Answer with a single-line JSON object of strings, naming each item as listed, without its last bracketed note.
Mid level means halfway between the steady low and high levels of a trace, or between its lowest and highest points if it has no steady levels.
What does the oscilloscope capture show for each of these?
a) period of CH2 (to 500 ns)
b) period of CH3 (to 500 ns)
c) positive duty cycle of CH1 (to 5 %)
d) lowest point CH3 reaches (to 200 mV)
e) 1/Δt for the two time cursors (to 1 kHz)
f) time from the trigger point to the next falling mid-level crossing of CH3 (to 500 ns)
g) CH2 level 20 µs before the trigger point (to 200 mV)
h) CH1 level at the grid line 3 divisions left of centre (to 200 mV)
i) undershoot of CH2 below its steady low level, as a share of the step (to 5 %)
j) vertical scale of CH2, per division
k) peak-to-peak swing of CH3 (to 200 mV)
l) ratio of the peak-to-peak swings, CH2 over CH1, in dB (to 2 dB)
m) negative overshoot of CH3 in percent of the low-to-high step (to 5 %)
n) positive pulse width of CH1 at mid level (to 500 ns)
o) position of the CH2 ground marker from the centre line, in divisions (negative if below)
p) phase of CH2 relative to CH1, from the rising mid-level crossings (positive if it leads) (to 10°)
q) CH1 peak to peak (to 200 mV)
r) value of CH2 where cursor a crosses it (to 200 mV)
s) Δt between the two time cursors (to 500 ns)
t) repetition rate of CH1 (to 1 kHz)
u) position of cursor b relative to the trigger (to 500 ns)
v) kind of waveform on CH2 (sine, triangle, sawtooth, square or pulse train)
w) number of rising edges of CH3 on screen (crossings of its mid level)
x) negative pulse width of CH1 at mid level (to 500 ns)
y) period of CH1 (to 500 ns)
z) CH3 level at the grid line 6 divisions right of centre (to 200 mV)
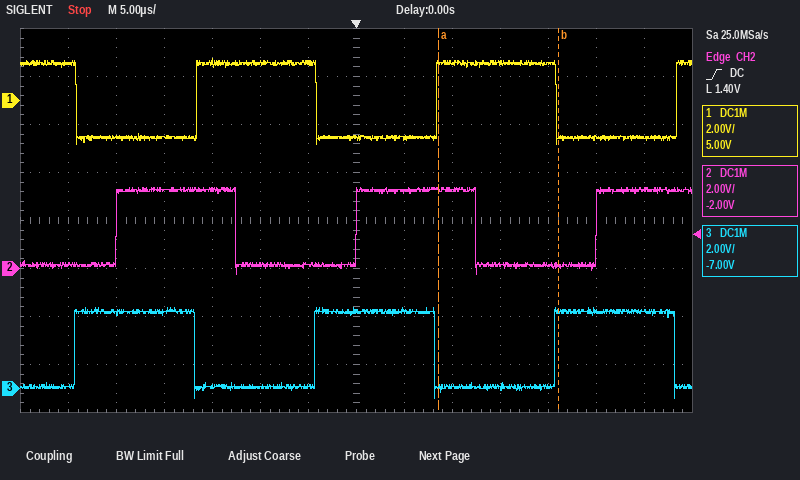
{"period of CH2": "25.0 µs", "period of CH3": "25.0 µs", "positive duty cycle of CH1": "50 %", "lowest point CH3 reaches": "-400 mV", "1/Δt for the two time cursors": "80 kHz", "time from the trigger point to the next falling mid-level crossing of CH3": "8.0 µs", "CH2 level 20 µs before the trigger point": "3.2 V", "CH1 level at the grid line 3 divisions left of centre": "1.6 V", "undershoot of CH2 below its steady low level, as a share of the step": "10 %", "vertical scale of CH2, per division": "2 V", "peak-to-peak swing of CH3": "3.8 V", "ratio of the peak-to-peak swings, CH2 over CH1, in dB": "0 dB", "negative overshoot of CH3 in percent of the low-to-high step": "15 %", "positive pulse width of CH1 at mid level": "12.5 µs", "position of the CH2 ground marker from the centre line, in divisions": "-1.0 div", "phase of CH2 relative to CH1, from the rising mid-level crossings (positive if it leads)": "+120°", "CH1 peak to peak": "3.6 V", "value of CH2 where cursor a crosses it": "3.2 V", "Δt between the two time cursors": "12.5 µs", "repetition rate of CH1": "40 kHz", "position of cursor b relative to the trigger": "+21.0 µs", "kind of waveform on CH2": "square", "number of rising edges of CH3 on screen": "3", "negative pulse width of CH1 at mid level": "12.5 µs", "period of CH1": "25.0 µs", "CH3 level at the grid line 6 divisions right of centre": "3.2 V"}
